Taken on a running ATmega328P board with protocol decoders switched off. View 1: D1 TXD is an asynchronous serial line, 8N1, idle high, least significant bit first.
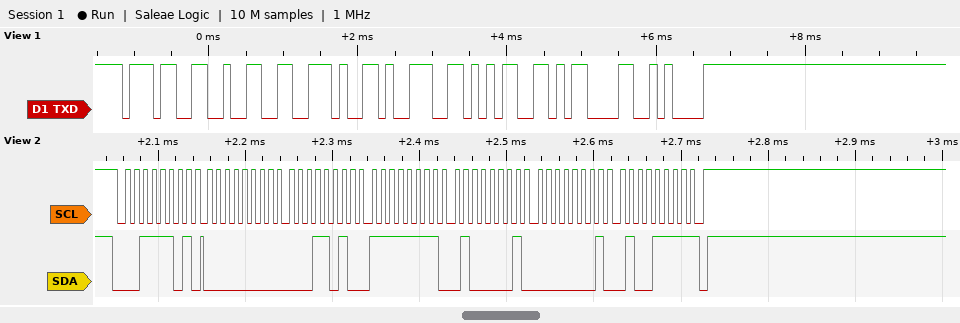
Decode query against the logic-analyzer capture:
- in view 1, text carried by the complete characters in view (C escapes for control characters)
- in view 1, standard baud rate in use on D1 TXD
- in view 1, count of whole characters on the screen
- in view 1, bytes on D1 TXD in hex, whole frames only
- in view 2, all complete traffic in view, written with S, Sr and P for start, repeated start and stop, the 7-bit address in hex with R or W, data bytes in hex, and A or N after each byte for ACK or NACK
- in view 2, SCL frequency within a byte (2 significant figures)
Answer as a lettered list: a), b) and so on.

a) "72.95\r\n"
b) 9600 baud
c) 7
d) 0x37 0x32 0x2E 0x39 0x35 0x0D 0x0A
e) S 1ER A 00 A 1A A FF A 41 A 01 A 4F N P
f) 100 kHz
